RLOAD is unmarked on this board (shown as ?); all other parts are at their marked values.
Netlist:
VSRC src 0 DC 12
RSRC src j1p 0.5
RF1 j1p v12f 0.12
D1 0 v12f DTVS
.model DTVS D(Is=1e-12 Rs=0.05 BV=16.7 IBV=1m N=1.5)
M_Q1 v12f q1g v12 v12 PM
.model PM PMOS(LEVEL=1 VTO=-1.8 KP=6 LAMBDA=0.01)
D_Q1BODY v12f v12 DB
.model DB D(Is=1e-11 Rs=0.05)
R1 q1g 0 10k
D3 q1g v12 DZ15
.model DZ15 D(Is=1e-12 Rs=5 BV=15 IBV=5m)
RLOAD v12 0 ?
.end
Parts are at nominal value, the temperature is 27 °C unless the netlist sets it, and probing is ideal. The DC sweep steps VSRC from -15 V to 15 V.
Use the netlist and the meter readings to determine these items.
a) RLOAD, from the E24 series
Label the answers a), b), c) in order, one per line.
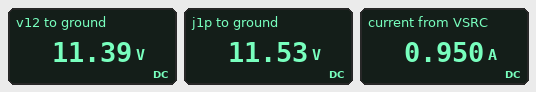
a) 12 Ω
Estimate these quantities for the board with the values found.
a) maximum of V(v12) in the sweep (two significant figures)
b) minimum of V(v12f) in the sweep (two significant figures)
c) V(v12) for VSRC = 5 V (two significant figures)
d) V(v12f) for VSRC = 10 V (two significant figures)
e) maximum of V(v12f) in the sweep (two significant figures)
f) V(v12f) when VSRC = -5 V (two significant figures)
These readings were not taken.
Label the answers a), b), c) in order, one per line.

a) 14 V
b) -2.2 V
c) 4.7 V
d) 9.5 V
e) 14 V
f) -1.4 V
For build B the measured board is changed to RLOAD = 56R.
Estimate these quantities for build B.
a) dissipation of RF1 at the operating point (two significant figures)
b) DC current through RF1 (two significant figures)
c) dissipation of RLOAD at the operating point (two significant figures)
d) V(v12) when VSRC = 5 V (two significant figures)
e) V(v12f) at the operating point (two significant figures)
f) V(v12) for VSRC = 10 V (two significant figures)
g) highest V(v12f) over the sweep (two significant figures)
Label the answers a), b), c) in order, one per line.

a) 5.4 mW
b) 210 mA
c) 2.5 W
d) 4.9 V
e) 12 V
f) 9.9 V
g) 15 V
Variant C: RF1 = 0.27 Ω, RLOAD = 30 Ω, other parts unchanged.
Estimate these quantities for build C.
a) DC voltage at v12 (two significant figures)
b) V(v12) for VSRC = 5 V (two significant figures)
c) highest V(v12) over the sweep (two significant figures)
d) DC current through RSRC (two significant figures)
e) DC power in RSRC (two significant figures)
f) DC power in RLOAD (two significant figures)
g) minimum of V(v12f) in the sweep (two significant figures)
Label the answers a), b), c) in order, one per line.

a) 12 V
b) 4.9 V
c) 15 V
d) 390 mA
e) 76 mW
f) 4.6 W
g) -2.0 V
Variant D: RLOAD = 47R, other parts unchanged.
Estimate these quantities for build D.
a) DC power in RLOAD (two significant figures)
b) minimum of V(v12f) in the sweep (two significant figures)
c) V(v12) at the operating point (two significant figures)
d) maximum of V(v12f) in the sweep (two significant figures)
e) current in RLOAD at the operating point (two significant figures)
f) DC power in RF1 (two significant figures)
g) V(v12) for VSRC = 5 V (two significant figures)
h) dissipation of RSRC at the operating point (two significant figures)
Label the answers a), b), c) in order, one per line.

a) 3.0 W
b) -2.2 V
c) 12 V
d) 15 V
e) 250 mA
f) 7.6 mW
g) 4.9 V
h) 32 mW
